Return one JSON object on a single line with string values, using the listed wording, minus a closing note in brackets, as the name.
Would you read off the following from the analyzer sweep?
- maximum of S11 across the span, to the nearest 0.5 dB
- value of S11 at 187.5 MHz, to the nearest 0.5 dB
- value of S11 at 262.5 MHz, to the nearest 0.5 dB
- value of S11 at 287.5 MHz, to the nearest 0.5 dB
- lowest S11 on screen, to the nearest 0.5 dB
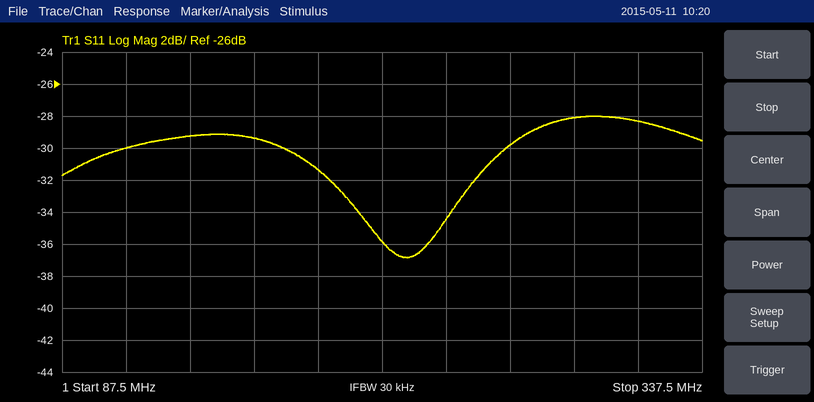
{"maximum of S11 across the span, to the nearest 0.5 dB": "-28.0 dB", "value of S11 at 187.5 MHz, to the nearest 0.5 dB": "-31.5 dB", "value of S11 at 262.5 MHz, to the nearest 0.5 dB": "-30.0 dB", "value of S11 at 287.5 MHz, to the nearest 0.5 dB": "-28.0 dB", "lowest S11 on screen, to the nearest 0.5 dB": "-37.0 dB"}
